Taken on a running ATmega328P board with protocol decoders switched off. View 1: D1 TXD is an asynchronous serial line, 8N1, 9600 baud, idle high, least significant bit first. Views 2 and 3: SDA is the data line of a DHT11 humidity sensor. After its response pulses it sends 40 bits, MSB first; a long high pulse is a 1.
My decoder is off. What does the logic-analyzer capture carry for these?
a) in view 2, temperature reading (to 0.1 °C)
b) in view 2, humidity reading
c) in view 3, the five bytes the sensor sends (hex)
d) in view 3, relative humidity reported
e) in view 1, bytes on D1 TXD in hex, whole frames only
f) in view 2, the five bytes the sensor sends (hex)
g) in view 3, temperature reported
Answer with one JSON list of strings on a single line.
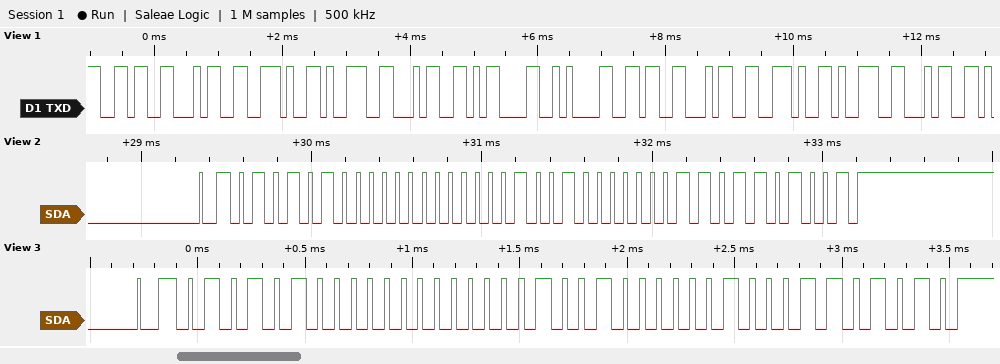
["18.3 °C", "84 %", "54 00 12 04 6A", "84 %", "36 34 2E 39 34 0D 0A 36 34 2E 39 34", "54 00 12 03 69", "18.4 °C"]
